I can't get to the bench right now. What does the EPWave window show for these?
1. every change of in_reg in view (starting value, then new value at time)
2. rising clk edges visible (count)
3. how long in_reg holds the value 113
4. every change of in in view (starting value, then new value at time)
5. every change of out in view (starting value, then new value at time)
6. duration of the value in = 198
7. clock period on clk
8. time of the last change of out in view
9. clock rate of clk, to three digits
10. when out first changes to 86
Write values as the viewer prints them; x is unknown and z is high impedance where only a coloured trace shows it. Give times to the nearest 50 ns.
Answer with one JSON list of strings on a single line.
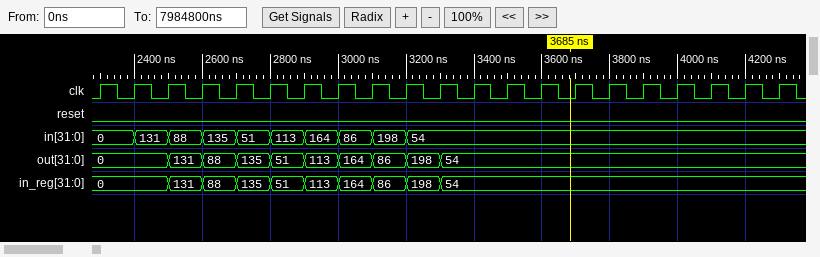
["0, 131 at 2500 ns, 88 at 2600 ns, 135 at 2700 ns, 51 at 2800 ns, 113 at 2900 ns, 164 at 3000 ns, 86 at 3100 ns, 198 at 3200 ns, 54 at 3300 ns", "21", "100 ns", "0, 131 at 2400 ns, 88 at 2500 ns, 135 at 2600 ns, 51 at 2700 ns, 113 at 2800 ns, 164 at 2900 ns, 86 at 3000 ns, 198 at 3100 ns, 54 at 3200 ns", "0, 131 at 2500 ns, 88 at 2600 ns, 135 at 2700 ns, 51 at 2800 ns, 113 at 2900 ns, 164 at 3000 ns, 86 at 3100 ns, 198 at 3200 ns, 54 at 3300 ns", "100 ns", "100 ns", "3300 ns", "10.0 MHz", "3100 ns"]
